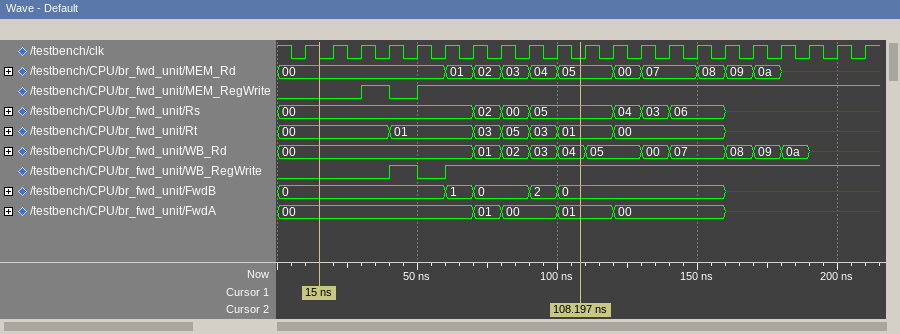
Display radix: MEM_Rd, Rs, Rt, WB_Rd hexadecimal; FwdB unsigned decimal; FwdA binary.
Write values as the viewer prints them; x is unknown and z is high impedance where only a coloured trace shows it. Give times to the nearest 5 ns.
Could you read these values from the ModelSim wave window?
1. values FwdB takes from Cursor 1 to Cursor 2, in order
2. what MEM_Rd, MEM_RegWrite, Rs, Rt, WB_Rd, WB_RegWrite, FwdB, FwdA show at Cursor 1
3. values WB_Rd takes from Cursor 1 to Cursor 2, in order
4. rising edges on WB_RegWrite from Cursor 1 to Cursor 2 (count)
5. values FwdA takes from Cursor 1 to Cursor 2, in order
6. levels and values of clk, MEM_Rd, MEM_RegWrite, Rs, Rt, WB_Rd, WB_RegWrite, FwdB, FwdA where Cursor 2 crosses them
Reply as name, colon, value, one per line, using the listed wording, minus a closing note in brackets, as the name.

values FwdB takes from Cursor 1 to Cursor 2, in order: 0, 1, 0, 2, 0
what MEM_Rd, MEM_RegWrite, Rs, Rt, WB_Rd, WB_RegWrite, FwdB, FwdA show at Cursor 1: MEM_Rd=00, MEM_RegWrite=0, Rs=00, Rt=00, WB_Rd=00, WB_RegWrite=0, FwdB=0, FwdA=00
values WB_Rd takes from Cursor 1 to Cursor 2, in order: 00, 01, 02, 03, 04
rising edges on WB_RegWrite from Cursor 1 to Cursor 2: 2
values FwdA takes from Cursor 1 to Cursor 2, in order: 00, 01, 00, 01
levels and values of clk, MEM_Rd, MEM_RegWrite, Rs, Rt, WB_Rd, WB_RegWrite, FwdB, FwdA where Cursor 2 crosses them: clk=0, MEM_Rd=05, MEM_RegWrite=1, Rs=05, Rt=01, WB_Rd=04, WB_RegWrite=1, FwdB=0, FwdA=01
